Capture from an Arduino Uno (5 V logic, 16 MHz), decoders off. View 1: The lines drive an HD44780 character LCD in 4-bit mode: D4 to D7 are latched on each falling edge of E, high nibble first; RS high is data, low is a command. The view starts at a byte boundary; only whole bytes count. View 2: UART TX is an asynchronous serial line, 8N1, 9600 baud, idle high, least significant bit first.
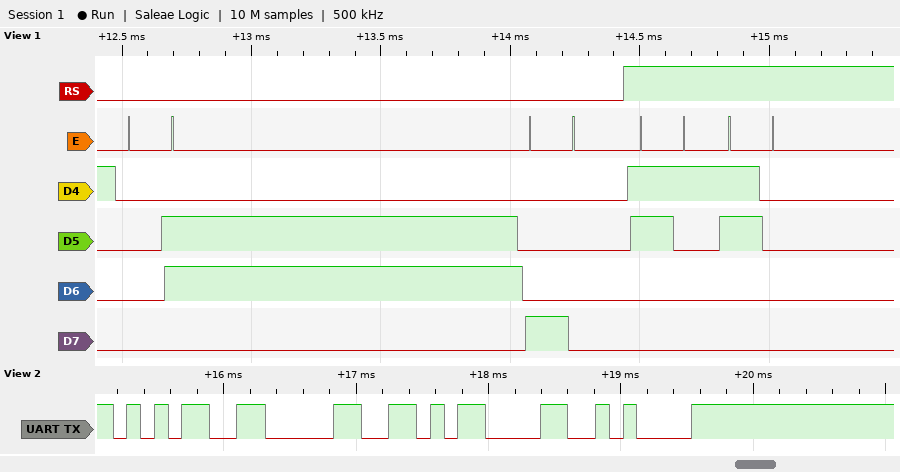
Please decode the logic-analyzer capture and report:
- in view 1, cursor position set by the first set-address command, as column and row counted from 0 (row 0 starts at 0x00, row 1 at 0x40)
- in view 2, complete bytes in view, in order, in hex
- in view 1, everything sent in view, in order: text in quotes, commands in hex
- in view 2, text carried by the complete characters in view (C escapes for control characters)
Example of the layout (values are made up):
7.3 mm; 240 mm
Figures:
column 0, row 0; 35 30 0D 0A; 0x06 0x80 "10"; "50\r\n"
